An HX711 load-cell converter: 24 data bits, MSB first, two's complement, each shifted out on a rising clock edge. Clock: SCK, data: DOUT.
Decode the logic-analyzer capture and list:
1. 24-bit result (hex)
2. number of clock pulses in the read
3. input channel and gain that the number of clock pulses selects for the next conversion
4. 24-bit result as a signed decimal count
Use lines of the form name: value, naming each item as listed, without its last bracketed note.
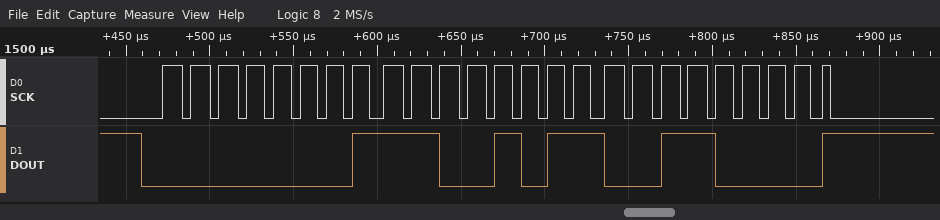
24-bit result: 0x01CB30
number of clock pulses in the read: 25
input channel and gain that the number of clock pulses selects for the next conversion: channel A, gain 128
24-bit result as a signed decimal count: 117552
